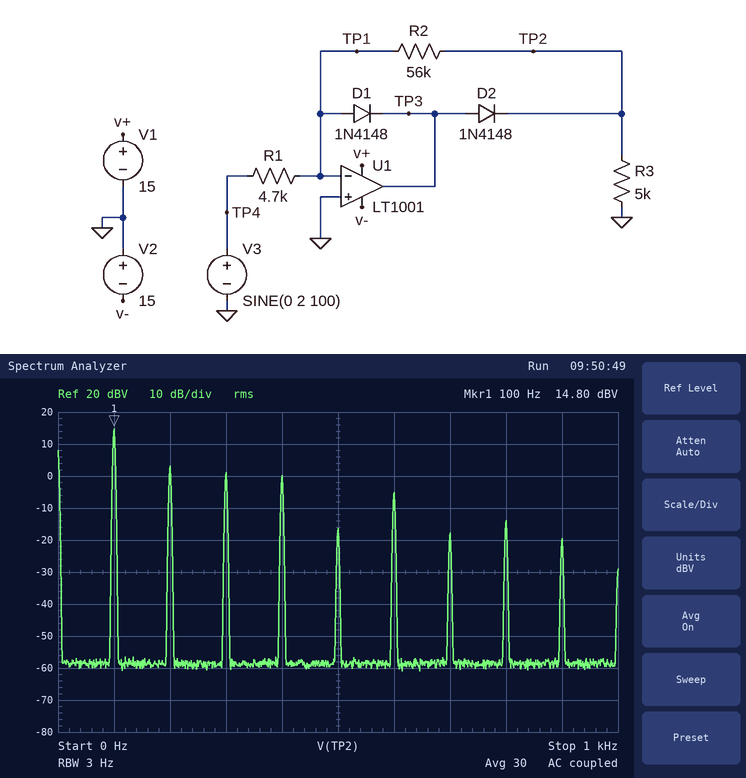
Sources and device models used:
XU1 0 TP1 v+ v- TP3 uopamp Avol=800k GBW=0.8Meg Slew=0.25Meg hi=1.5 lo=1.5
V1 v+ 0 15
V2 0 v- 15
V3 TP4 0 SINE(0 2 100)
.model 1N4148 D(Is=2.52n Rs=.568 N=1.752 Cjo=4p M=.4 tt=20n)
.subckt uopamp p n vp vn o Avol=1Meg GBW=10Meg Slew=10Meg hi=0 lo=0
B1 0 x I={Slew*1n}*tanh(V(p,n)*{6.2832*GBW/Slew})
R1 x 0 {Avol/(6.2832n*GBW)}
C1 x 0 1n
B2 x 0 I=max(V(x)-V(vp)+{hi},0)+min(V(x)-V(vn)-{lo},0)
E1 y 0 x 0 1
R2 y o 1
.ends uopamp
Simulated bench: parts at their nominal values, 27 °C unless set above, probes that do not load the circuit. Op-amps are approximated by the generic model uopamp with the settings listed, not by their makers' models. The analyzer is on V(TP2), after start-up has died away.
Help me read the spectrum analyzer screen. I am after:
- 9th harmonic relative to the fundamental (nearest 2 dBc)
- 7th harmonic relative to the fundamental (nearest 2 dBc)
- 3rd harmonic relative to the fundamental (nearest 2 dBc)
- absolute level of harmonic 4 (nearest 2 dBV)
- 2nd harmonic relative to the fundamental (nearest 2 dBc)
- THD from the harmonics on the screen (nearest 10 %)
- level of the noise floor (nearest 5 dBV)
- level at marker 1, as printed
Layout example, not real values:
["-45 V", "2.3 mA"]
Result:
["-34 dBc", "-32 dBc", "-14 dBc", "0 dBV", "-12 dBc", "40 %", "-60 dBV", "14.80 dBV"]
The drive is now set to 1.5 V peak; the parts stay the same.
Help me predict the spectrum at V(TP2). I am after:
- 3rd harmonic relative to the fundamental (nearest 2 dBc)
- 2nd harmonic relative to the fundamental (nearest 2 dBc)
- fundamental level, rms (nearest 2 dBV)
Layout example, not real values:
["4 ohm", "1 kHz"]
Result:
["-18 dBc", "-10 dBc", "14 dBV"]
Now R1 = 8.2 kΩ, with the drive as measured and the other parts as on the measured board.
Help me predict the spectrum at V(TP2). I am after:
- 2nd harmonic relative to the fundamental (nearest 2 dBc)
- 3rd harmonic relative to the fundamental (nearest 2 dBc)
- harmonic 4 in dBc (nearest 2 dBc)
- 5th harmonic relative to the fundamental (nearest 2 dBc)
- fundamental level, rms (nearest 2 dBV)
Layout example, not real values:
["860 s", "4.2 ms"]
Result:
["-8 dBc", "-36 dBc", "-20 dBc", "-38 dBc", "14 dBV"]
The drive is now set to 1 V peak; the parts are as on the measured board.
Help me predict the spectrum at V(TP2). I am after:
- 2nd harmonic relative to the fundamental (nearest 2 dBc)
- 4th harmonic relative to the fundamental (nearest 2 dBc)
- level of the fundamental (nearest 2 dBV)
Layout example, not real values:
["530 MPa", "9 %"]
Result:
["-8 dBc", "-22 dBc", "12 dBV"]
